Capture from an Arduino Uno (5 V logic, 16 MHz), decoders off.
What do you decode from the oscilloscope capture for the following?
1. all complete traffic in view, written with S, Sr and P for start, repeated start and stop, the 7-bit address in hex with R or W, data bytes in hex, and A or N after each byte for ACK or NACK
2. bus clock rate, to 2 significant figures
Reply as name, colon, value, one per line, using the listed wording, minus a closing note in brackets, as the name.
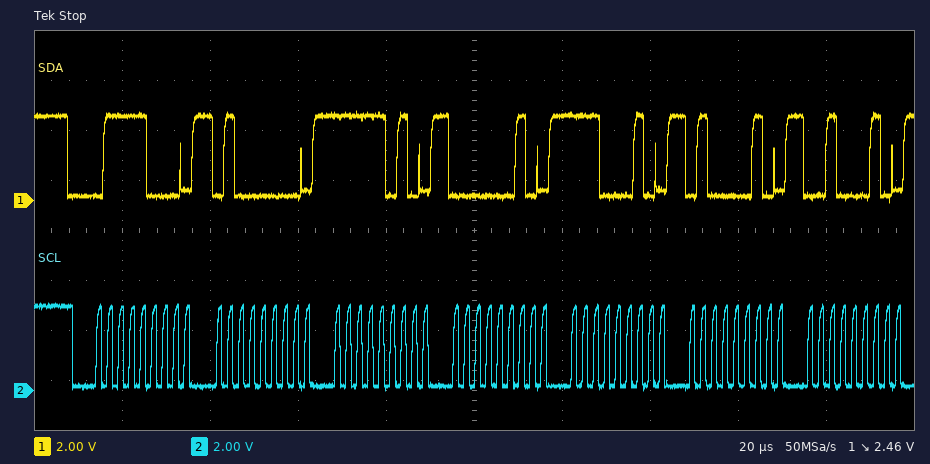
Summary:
all complete traffic in view, written with S, Sr and P for start, repeated start and stop, the 7-bit address in hex with R or W, data bytes in hex, and A or N after each byte for ACK or NACK: S 3CW A 40 A FA A 02 A E2 A 42 A 22 A
bus clock rate, to 2 significant figures: 400 kHz
